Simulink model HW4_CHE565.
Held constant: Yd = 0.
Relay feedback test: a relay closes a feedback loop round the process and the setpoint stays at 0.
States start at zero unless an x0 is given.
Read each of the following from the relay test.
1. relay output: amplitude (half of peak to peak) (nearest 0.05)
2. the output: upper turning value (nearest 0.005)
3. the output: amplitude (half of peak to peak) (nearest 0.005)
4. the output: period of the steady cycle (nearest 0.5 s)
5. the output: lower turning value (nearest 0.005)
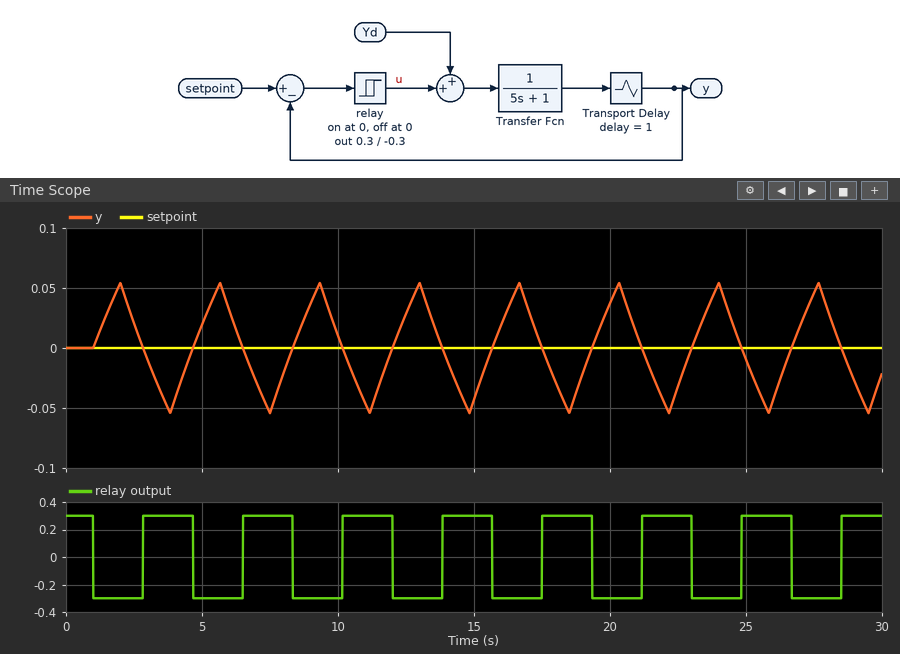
0.30
0.055
0.055
3.5 s
-0.055
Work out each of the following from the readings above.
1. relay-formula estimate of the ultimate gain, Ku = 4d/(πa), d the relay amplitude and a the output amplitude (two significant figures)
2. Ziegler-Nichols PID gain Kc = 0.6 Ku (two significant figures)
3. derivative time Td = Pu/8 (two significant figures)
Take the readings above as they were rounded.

6.9
4.1
0.44 s
